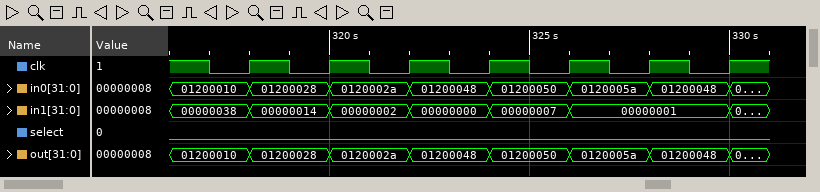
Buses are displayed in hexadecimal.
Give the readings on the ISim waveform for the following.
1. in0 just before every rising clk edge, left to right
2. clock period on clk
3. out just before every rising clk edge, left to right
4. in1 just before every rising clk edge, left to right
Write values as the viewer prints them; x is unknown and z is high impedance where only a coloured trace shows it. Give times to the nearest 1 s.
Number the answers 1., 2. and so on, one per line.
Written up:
1. 01200010, 01200028, 0120002a, 01200048, 01200050, 0120005a, 01200048
2. 2 s
3. 01200010, 01200028, 0120002a, 01200048, 01200050, 0120005a, 01200048
4. 00000038, 00000014, 00000002, 00000000, 00000007, 00000001, 00000001
